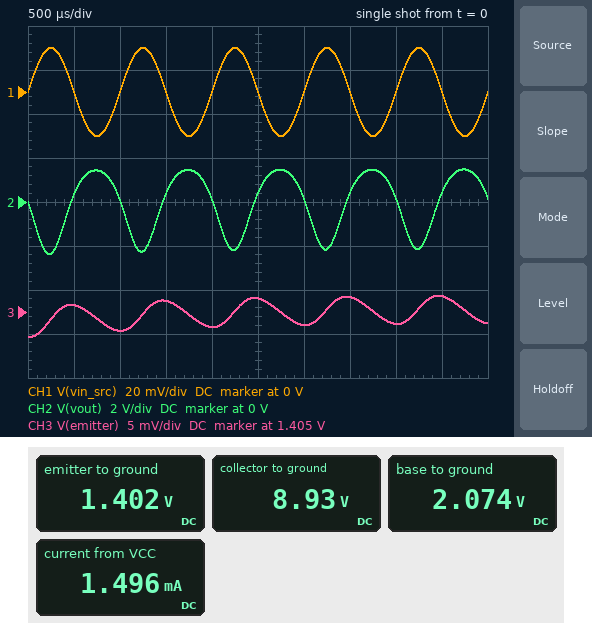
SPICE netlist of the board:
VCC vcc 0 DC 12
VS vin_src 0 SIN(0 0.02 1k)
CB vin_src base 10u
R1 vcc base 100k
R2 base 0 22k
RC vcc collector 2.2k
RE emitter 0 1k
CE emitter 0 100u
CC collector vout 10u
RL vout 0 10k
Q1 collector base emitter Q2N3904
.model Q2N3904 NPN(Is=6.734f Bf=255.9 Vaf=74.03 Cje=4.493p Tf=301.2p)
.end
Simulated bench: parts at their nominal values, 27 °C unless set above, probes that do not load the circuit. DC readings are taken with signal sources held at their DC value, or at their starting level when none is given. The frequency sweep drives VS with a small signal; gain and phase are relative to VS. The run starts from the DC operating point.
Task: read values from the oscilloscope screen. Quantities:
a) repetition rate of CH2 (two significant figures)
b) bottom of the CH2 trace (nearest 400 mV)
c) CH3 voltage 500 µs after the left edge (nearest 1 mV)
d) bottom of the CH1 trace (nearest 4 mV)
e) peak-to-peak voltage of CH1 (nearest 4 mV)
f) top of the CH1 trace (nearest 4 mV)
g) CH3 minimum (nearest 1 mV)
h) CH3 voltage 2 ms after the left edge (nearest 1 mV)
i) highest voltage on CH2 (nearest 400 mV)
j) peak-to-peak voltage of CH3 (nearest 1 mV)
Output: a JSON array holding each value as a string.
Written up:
["1.0 kHz", "-2.4 V", "1.406 V", "-20 mV", "40 mV", "20 mV", "1.402 V", "1.403 V", "1.6 V", "5 mV"]
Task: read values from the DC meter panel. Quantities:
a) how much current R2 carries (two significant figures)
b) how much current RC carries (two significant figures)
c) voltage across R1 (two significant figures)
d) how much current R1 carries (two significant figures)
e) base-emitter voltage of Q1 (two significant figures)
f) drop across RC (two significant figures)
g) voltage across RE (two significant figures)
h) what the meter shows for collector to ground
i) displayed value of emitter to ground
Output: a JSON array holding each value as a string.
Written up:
["94 µA", "1.4 mA", "9.9 V", "99 µA", "670 mV", "3.1 V", "1.4 V", "8.93 V", "1.402 V"]
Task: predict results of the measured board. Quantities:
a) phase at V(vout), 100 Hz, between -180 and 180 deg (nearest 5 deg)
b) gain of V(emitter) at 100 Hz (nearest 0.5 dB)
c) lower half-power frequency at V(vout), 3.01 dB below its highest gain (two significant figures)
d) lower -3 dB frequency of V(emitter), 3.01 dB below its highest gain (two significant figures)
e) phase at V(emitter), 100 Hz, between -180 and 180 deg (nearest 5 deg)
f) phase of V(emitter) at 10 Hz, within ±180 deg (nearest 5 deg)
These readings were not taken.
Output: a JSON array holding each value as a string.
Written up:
["-140 deg", "-4.0 dB", "88 Hz", "890 mHz", "-50 deg", "0 deg"]
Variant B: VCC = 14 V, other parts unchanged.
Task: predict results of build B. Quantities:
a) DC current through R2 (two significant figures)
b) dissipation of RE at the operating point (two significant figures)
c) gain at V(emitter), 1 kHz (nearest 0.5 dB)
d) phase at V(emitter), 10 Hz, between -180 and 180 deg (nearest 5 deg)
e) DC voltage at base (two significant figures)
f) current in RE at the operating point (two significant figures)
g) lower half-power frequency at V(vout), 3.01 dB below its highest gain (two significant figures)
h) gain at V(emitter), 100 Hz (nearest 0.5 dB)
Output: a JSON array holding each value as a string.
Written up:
["110 µA", "3.0 mW", "-20.0 dB", "0 deg", "2.4 V", "1.7 mA", "110 Hz", "-3.0 dB"]
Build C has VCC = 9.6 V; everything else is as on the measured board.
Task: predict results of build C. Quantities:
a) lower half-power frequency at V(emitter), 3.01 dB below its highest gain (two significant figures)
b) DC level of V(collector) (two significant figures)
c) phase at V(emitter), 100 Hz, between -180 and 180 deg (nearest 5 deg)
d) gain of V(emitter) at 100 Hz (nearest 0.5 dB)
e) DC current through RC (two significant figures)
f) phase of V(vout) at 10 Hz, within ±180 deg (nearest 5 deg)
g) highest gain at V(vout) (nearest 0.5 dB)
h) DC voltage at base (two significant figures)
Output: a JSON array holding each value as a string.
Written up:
["880 mHz", "7.4 V", "-55 deg", "-6.0 dB", "1.0 mA", "-95 deg", "36.5 dB", "1.7 V"]
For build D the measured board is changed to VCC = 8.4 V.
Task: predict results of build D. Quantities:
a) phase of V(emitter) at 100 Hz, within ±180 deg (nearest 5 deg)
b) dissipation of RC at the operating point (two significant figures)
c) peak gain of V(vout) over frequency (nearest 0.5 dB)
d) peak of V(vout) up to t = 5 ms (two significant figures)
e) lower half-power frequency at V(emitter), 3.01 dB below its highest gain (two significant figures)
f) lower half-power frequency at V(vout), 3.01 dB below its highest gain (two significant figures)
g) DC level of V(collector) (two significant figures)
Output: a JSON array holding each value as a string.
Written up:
["-60 deg", "1.4 mW", "35.0 dB", "850 mV", "880 mHz", "52 Hz", "6.6 V"]
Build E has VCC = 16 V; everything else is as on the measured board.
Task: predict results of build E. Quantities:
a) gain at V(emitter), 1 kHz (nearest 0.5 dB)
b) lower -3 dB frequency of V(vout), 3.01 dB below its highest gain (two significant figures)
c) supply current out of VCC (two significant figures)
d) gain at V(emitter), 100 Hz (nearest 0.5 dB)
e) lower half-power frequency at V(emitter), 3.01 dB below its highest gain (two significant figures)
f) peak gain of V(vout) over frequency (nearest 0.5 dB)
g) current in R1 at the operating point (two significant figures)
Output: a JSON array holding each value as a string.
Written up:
["-18.5 dB", "130 Hz", "2.2 mA", "-2.5 dB", "900 mHz", "43.0 dB", "130 µA"]
